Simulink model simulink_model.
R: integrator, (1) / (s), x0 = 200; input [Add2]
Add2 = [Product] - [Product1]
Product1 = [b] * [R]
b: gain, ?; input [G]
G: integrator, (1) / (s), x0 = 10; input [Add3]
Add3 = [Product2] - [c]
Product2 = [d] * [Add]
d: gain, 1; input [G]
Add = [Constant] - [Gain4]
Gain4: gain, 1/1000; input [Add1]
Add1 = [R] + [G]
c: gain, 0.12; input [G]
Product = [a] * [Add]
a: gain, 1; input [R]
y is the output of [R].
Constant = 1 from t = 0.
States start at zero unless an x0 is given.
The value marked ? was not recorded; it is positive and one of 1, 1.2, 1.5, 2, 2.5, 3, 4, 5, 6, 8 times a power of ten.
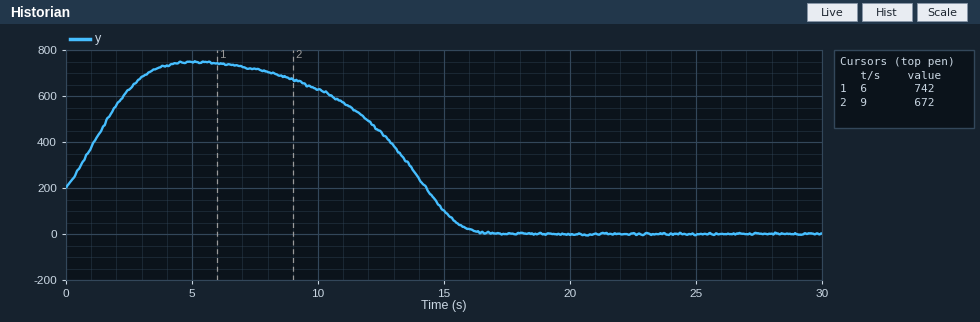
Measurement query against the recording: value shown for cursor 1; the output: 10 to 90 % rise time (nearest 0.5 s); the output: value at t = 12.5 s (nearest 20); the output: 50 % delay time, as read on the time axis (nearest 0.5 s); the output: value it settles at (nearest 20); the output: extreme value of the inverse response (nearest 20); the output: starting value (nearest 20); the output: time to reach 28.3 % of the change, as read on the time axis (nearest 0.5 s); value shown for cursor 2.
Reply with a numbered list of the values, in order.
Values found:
1. 742
2. 1.5 s
3. 440
4. 15.0 s
5. 0
6. 740
7. 200
8. 14.5 s
9. 672
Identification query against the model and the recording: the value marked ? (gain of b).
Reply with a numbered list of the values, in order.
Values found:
1. 0.005
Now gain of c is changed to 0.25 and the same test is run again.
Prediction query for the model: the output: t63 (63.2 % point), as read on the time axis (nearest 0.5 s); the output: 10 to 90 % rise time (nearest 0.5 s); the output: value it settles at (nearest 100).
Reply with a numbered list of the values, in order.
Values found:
1. 3.0 s
2. 8.5 s
3. 1000
